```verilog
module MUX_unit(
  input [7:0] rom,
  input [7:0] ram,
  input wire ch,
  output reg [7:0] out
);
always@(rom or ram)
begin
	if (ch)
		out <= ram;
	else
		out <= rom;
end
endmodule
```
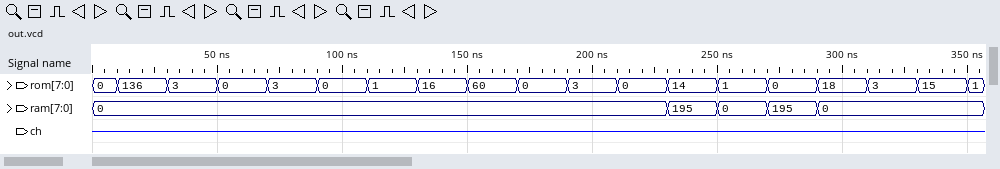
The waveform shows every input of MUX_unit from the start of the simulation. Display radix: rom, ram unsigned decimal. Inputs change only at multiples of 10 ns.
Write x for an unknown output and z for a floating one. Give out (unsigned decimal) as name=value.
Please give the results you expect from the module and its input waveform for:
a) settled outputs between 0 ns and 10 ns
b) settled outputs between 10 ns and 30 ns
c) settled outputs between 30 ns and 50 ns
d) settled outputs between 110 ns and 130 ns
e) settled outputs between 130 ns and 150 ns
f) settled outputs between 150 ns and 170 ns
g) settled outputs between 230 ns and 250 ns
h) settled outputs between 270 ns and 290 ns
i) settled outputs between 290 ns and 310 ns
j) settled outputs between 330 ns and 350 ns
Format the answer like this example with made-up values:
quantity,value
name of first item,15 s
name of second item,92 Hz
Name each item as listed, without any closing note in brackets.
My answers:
quantity,value
settled outputs between 0 ns and 10 ns,out=0
settled outputs between 10 ns and 30 ns,out=136
settled outputs between 30 ns and 50 ns,out=3
settled outputs between 110 ns and 130 ns,out=1
settled outputs between 130 ns and 150 ns,out=16
settled outputs between 150 ns and 170 ns,out=60
settled outputs between 230 ns and 250 ns,out=14
settled outputs between 270 ns and 290 ns,out=0
settled outputs between 290 ns and 310 ns,out=18
settled outputs between 330 ns and 350 ns,out=15
